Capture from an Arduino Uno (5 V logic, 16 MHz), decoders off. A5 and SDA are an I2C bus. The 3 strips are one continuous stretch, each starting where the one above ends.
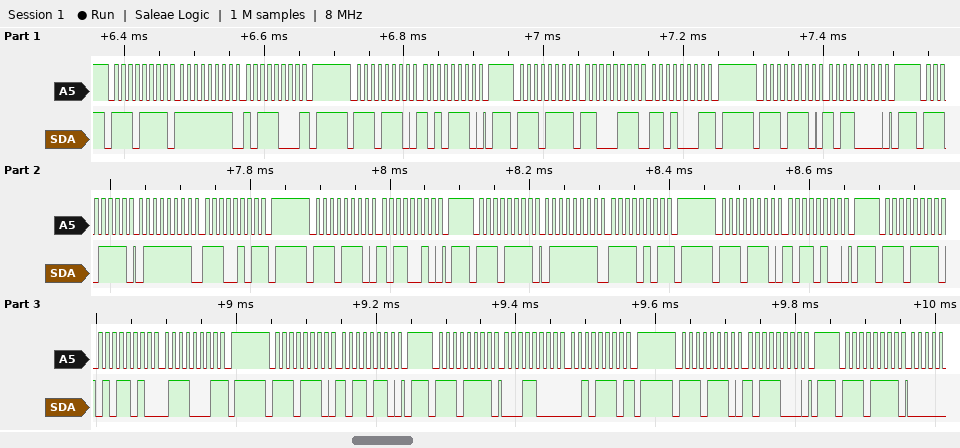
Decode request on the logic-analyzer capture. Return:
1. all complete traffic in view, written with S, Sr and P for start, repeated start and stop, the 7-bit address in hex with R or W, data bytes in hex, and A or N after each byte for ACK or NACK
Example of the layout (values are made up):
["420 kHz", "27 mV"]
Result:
["S 77R A FF A B8 N P S 77W A AE A P S 77R A C7 A D1 N P S 77W A B0 A P S 77R A 7F A E5 N P S 77W A B2 A P S 77R A 7F A F5 N P S 77W A B4 A P S 77R A 5A A 71 N P S 77W A B6 A P S 77R A 18 A 2E N P S 77W A B8 A P S 77R A"]
